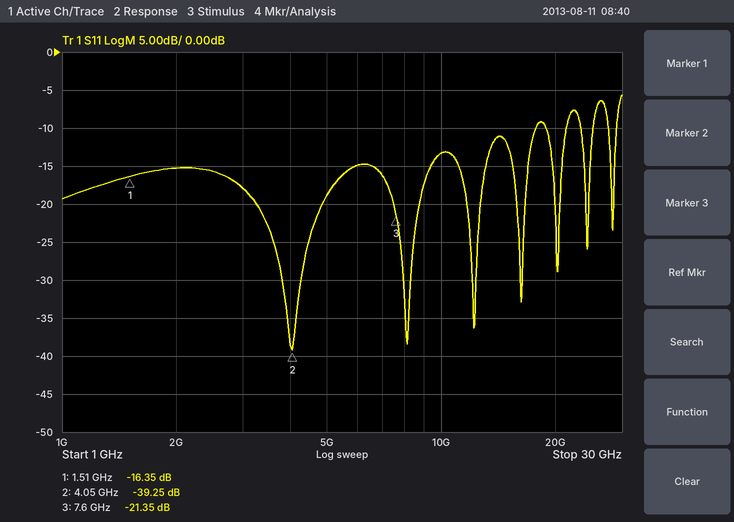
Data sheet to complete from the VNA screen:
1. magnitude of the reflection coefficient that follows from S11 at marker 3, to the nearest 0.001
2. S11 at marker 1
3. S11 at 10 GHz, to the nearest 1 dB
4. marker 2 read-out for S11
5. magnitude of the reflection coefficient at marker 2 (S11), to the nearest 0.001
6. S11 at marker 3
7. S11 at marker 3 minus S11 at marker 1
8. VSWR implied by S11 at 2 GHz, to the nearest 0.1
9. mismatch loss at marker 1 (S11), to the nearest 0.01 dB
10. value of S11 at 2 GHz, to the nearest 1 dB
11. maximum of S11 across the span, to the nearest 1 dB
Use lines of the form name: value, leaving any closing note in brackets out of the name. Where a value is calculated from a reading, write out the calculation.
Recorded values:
magnitude of the reflection coefficient that follows from S11 at marker 3, to the nearest 0.001: 10^(-21.35/20) ≈ 0.086
S11 at marker 1: -16.35 dB
S11 at 10 GHz, to the nearest 1 dB: -13 dB
marker 2 read-out for S11: -39.25 dB
magnitude of the reflection coefficient at marker 2 (S11), to the nearest 0.001: 10^(-39.25/20) ≈ 0.011
S11 at marker 3: -21.35 dB
S11 at marker 3 minus S11 at marker 1: -21.35 − (-16.35) = -5.00 dB
VSWR implied by S11 at 2 GHz, to the nearest 0.1: |Γ| = 10^(-15/20) = 0.1778; VSWR = (1 + 0.1778)/(1 − 0.1778) ≈ 1.4
mismatch loss at marker 1 (S11), to the nearest 0.01 dB: −10 log10(1 − 10^(-16.35/10)) ≈ 0.10 dB
value of S11 at 2 GHz, to the nearest 1 dB: -15 dB
maximum of S11 across the span, to the nearest 1 dB: -6 dB
